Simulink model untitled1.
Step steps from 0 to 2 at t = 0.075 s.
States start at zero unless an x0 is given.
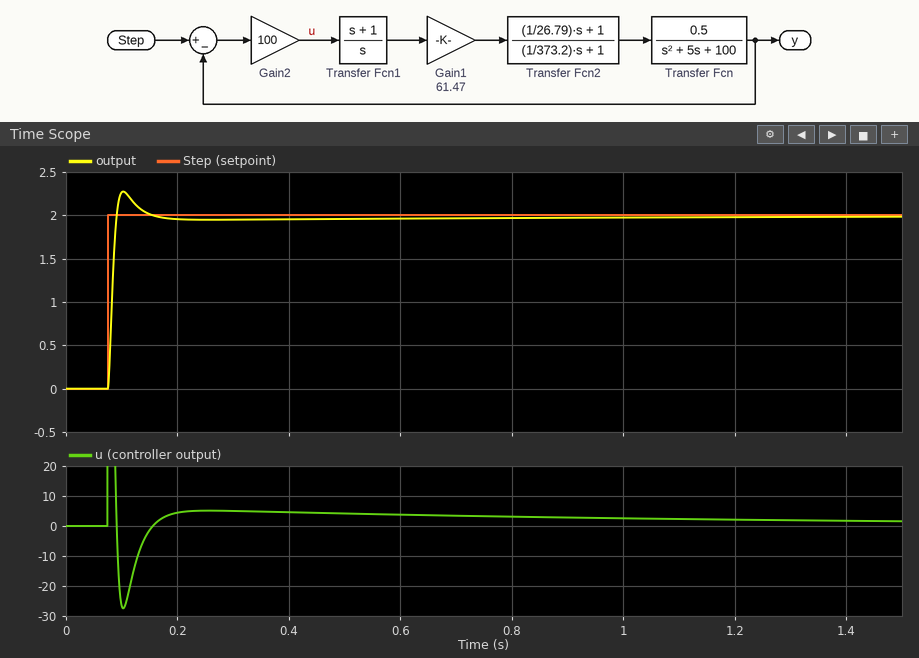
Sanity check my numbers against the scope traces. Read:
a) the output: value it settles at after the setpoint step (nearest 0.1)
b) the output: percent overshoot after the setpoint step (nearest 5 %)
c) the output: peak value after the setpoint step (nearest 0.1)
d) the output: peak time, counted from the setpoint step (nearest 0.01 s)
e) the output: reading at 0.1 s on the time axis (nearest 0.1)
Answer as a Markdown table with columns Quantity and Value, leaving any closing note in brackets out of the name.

| Quantity | Value |
|---|---|
| the output: value it settles at after the setpoint step | 2.0 |
| the output: percent overshoot after the setpoint step | 15 % |
| the output: peak value after the setpoint step | 2.3 |
| the output: peak time, counted from the setpoint step | 0.03 s |
| the output: reading at 0.1 s on the time axis | 2.3 |
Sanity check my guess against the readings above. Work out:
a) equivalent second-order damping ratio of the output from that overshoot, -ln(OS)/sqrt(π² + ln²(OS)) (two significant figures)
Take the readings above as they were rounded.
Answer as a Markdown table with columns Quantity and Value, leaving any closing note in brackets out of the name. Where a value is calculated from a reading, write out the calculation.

| Quantity | Value |
|---|---|
| equivalent second-order damping ratio of the output from that overshoot, -ln(OS)/sqrt(π² + ln²(OS)) | ln(0.15) = -1.897; 1.897 / sqrt(9.870 + 3.599) = 0.52 |
